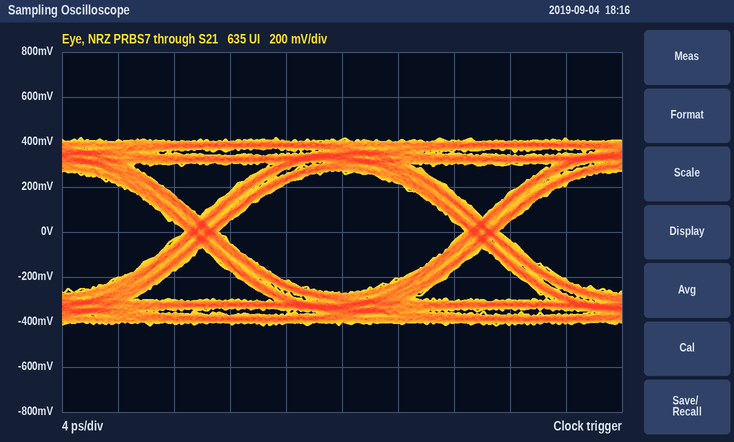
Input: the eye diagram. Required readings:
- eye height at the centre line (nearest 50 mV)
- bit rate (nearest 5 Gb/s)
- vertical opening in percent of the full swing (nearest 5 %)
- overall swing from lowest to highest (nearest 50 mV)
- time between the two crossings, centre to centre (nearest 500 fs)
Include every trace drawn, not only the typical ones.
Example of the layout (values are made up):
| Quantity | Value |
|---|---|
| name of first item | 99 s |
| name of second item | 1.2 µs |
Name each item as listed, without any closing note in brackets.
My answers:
| Quantity | Value |
|---|---|
| eye height at the centre line | 550 mV |
| bit rate | 50 Gb/s |
| vertical opening in percent of the full swing | 65 % |
| overall swing from lowest to highest | 850 mV |
| time between the two crossings, centre to centre | 20.0 ps |
